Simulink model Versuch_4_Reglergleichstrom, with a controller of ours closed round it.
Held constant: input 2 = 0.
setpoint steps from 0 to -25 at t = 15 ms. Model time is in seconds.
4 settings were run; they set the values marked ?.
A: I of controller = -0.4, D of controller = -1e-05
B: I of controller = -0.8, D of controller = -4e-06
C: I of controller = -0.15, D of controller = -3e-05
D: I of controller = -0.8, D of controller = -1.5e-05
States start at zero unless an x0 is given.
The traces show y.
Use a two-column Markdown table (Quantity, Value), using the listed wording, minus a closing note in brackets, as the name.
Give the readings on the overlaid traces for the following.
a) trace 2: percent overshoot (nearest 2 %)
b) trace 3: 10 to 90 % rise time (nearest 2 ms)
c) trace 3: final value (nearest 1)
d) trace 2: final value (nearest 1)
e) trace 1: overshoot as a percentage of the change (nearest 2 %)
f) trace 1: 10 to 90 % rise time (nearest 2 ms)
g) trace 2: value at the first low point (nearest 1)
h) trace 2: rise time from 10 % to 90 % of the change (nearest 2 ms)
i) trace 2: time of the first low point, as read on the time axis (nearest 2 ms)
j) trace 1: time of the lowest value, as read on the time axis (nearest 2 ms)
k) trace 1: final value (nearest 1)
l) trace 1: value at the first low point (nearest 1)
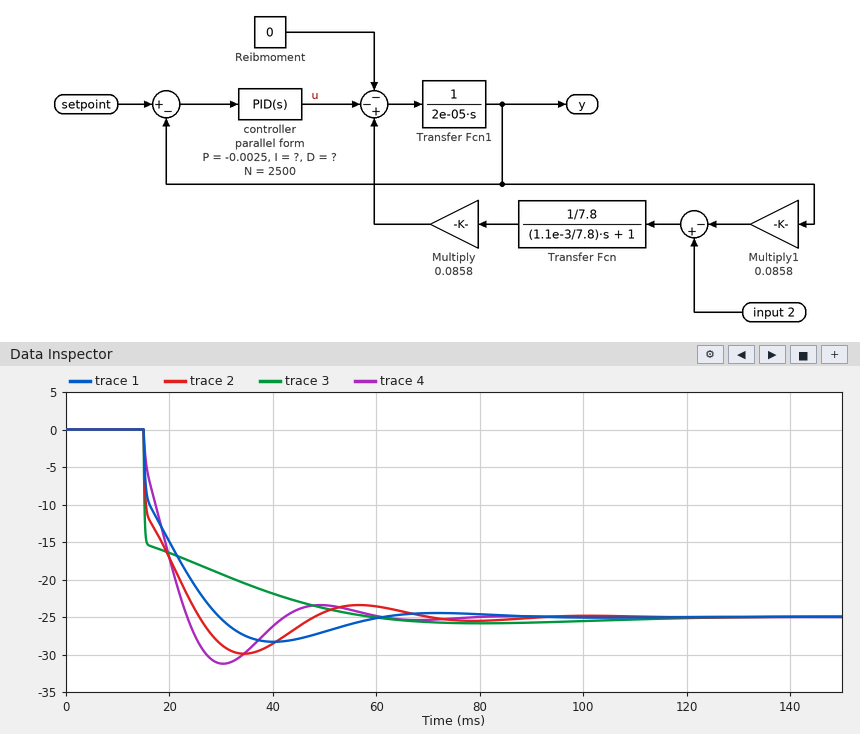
| Quantity | Value |
|---|---|
| trace 2: percent overshoot | 20 % |
| trace 3: 10 to 90 % rise time | 28 ms |
| trace 3: final value | -25 |
| trace 2: final value | -25 |
| trace 1: overshoot as a percentage of the change | 14 % |
| trace 1: 10 to 90 % rise time | 12 ms |
| trace 2: value at the first low point | -30 |
| trace 2: rise time from 10 % to 90 % of the change | 8 ms |
| trace 2: time of the first low point, as read on the time axis | 34 ms |
| trace 1: time of the lowest value, as read on the time axis | 40 ms |
| trace 1: final value | -25 |
| trace 1: value at the first low point | -28 |
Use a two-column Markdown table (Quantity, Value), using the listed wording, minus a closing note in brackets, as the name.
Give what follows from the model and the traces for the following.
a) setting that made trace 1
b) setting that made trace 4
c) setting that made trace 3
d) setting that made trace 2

| Quantity | Value |
|---|---|
| setting that made trace 1 | A |
| setting that made trace 4 | B |
| setting that made trace 3 | C |
| setting that made trace 2 | D |
